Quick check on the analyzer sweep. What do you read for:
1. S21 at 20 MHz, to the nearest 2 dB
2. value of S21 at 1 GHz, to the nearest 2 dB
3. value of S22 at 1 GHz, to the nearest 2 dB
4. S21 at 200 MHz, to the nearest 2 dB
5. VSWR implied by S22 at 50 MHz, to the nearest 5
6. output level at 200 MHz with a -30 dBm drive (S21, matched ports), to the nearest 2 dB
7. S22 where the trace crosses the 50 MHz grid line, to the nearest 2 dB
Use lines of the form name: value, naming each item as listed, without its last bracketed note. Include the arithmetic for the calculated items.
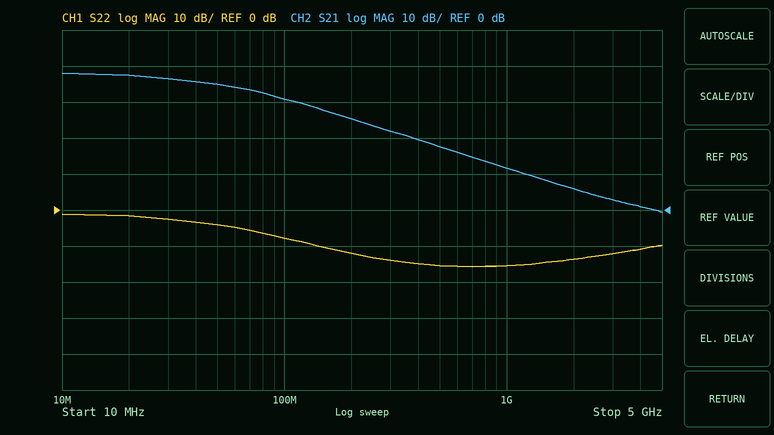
S21 at 20 MHz, to the nearest 2 dB: 38 dB
value of S21 at 1 GHz, to the nearest 2 dB: 12 dB
value of S22 at 1 GHz, to the nearest 2 dB: -16 dB
S21 at 200 MHz, to the nearest 2 dB: 26 dB
VSWR implied by S22 at 50 MHz, to the nearest 5: |Γ| = 10^(-4/20) = 0.6310; VSWR = (1 + 0.6310)/(1 − 0.6310) ≈ 4.42, so 5 to the nearest 5
output level at 200 MHz with a -30 dBm drive (S21, matched ports), to the nearest 2 dB: -30 dBm + (26 dB) = -4 dBm
S22 where the trace crosses the 50 MHz grid line, to the nearest 2 dB: -4 dB
